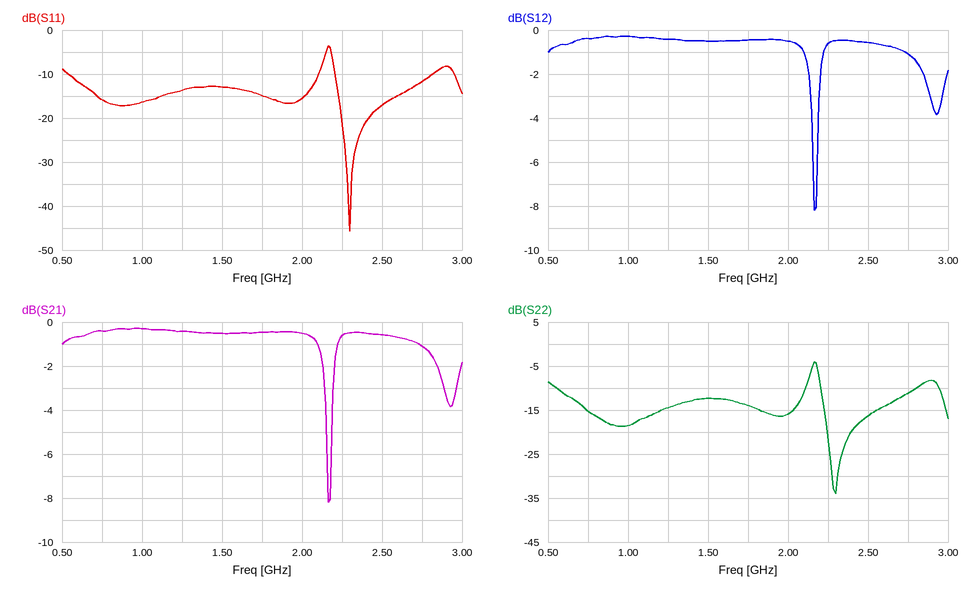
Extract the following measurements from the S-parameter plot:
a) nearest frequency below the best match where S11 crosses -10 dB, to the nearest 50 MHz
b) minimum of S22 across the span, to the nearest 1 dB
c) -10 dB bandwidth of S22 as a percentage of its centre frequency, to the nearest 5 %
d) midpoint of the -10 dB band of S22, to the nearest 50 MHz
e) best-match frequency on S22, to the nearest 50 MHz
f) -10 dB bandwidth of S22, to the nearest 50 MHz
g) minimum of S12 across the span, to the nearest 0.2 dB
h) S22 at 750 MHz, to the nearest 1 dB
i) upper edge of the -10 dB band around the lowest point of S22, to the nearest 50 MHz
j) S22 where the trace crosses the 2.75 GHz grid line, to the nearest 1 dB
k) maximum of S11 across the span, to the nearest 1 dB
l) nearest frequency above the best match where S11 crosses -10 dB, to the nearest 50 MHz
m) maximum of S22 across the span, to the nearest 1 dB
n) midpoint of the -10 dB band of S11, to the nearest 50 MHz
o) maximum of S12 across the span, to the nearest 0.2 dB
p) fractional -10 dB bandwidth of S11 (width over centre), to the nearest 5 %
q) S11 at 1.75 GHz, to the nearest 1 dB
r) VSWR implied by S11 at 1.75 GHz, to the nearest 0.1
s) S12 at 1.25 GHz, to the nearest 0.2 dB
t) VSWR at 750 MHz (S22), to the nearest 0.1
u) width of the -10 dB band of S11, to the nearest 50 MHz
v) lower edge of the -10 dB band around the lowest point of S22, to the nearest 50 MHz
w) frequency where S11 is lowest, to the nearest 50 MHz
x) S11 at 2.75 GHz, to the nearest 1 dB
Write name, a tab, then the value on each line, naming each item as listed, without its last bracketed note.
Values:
nearest frequency below the best match where S11 crosses -10 dB, to the nearest 50 MHz	2.20 GHz
minimum of S22 across the span, to the nearest 1 dB	-34 dB
-10 dB bandwidth of S22 as a percentage of its centre frequency, to the nearest 5 %	25 %
midpoint of the -10 dB band of S22, to the nearest 50 MHz	2.50 GHz
best-match frequency on S22, to the nearest 50 MHz	2.30 GHz
-10 dB bandwidth of S22, to the nearest 50 MHz	600 MHz
minimum of S12 across the span, to the nearest 0.2 dB	-8.2 dB
S22 at 750 MHz, to the nearest 1 dB	-15 dB
upper edge of the -10 dB band around the lowest point of S22, to the nearest 50 MHz	2.80 GHz
S22 where the trace crosses the 2.75 GHz grid line, to the nearest 1 dB	-11 dB
maximum of S11 across the span, to the nearest 1 dB	-4 dB
nearest frequency above the best match where S11 crosses -10 dB, to the nearest 50 MHz	2.80 GHz
maximum of S22 across the span, to the nearest 1 dB	-4 dB
midpoint of the -10 dB band of S11, to the nearest 50 MHz	2.50 GHz
maximum of S12 across the span, to the nearest 0.2 dB	-0.2 dB
fractional -10 dB bandwidth of S11 (width over centre), to the nearest 5 %	25 %
S11 at 1.75 GHz, to the nearest 1 dB	-15 dB
VSWR implied by S11 at 1.75 GHz, to the nearest 0.1	1.4
S12 at 1.25 GHz, to the nearest 0.2 dB	-0.4 dB
VSWR at 750 MHz (S22), to the nearest 0.1	1.4
width of the -10 dB band of S11, to the nearest 50 MHz	600 MHz
lower edge of the -10 dB band around the lowest point of S22, to the nearest 50 MHz	2.20 GHz
frequency where S11 is lowest, to the nearest 50 MHz	2.30 GHz
S11 at 2.75 GHz, to the nearest 1 dB	-12 dB
